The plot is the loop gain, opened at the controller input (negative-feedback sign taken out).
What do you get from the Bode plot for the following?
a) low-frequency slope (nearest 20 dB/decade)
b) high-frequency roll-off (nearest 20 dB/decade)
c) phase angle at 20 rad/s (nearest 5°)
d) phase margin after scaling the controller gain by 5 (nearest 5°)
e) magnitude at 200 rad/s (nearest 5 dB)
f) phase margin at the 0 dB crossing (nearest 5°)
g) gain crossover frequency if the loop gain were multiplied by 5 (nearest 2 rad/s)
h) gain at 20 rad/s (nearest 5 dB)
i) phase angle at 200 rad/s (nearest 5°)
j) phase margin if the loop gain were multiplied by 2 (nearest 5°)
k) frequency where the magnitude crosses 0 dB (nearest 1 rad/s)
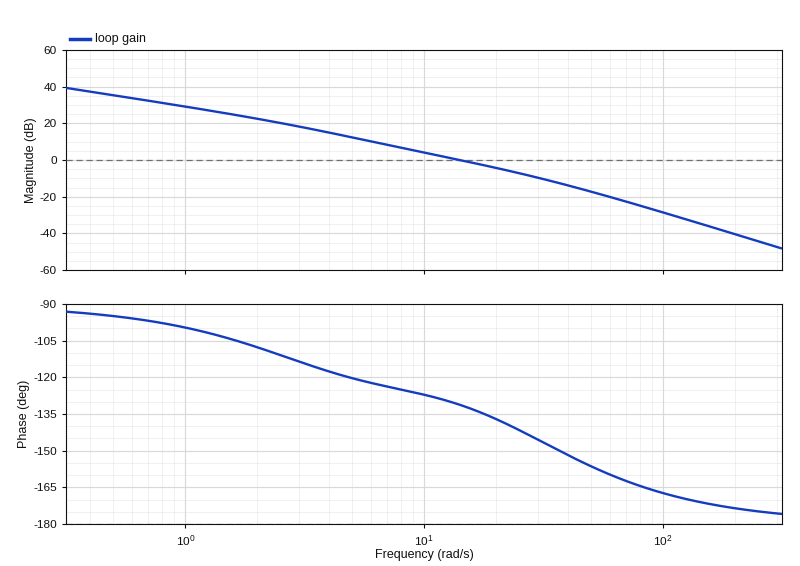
-20 dB/decade
-40 dB/decade
-135°
30°
-40 dB
50°
40 rad/s
-5 dB
-175°
40°
14 rad/s
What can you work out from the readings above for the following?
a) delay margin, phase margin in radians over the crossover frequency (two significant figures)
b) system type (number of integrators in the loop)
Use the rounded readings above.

0.062 s
1
